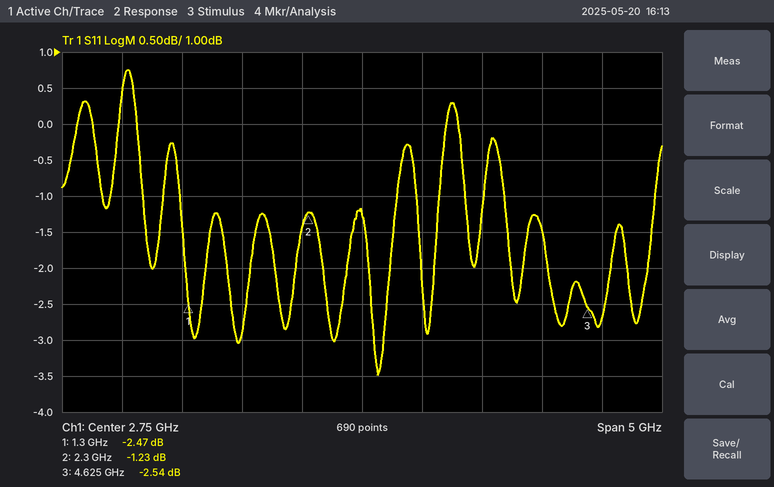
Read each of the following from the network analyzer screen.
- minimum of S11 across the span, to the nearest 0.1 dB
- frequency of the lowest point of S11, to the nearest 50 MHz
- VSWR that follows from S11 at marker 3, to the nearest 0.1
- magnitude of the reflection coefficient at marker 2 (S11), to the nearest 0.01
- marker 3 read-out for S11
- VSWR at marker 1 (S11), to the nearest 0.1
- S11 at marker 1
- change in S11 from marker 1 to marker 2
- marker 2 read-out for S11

-3.5 dB
2.90 GHz
6.9
0.87
-2.54 dB
7.1
-2.47 dB
1.24 dB
-1.23 dB
